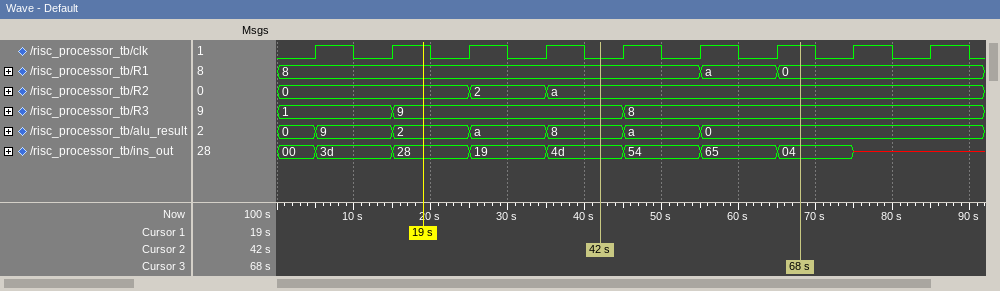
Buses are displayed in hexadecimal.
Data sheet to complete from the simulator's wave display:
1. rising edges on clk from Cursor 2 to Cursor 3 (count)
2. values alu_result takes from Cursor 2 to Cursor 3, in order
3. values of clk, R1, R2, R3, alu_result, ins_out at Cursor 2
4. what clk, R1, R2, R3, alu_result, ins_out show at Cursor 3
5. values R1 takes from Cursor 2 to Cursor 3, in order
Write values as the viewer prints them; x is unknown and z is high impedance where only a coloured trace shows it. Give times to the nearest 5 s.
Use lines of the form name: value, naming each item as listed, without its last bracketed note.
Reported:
rising edges on clk from Cursor 2 to Cursor 3: 3
values alu_result takes from Cursor 2 to Cursor 3, in order: 8, a, 0
values of clk, R1, R2, R3, alu_result, ins_out at Cursor 2: clk=0, R1=8, R2=a, R3=9, alu_result=8, ins_out=4d
what clk, R1, R2, R3, alu_result, ins_out show at Cursor 3: clk=1, R1=0, R2=a, R3=8, alu_result=0, ins_out=04
values R1 takes from Cursor 2 to Cursor 3, in order: 8, a, 0
